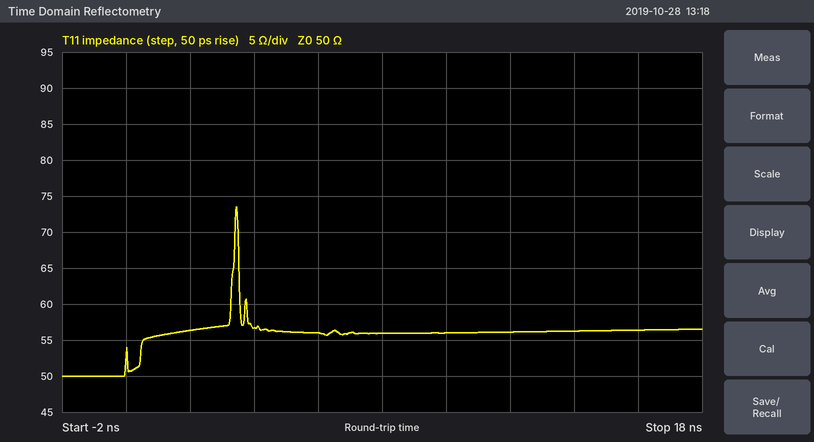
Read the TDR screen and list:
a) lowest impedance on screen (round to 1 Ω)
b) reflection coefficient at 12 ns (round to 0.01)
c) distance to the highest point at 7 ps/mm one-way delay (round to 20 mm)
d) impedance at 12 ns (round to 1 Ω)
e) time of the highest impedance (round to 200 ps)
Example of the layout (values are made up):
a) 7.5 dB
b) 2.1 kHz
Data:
a) 50 Ω
b) +0.06
c) 240 mm
d) 56 Ω
e) 3.4 ns
